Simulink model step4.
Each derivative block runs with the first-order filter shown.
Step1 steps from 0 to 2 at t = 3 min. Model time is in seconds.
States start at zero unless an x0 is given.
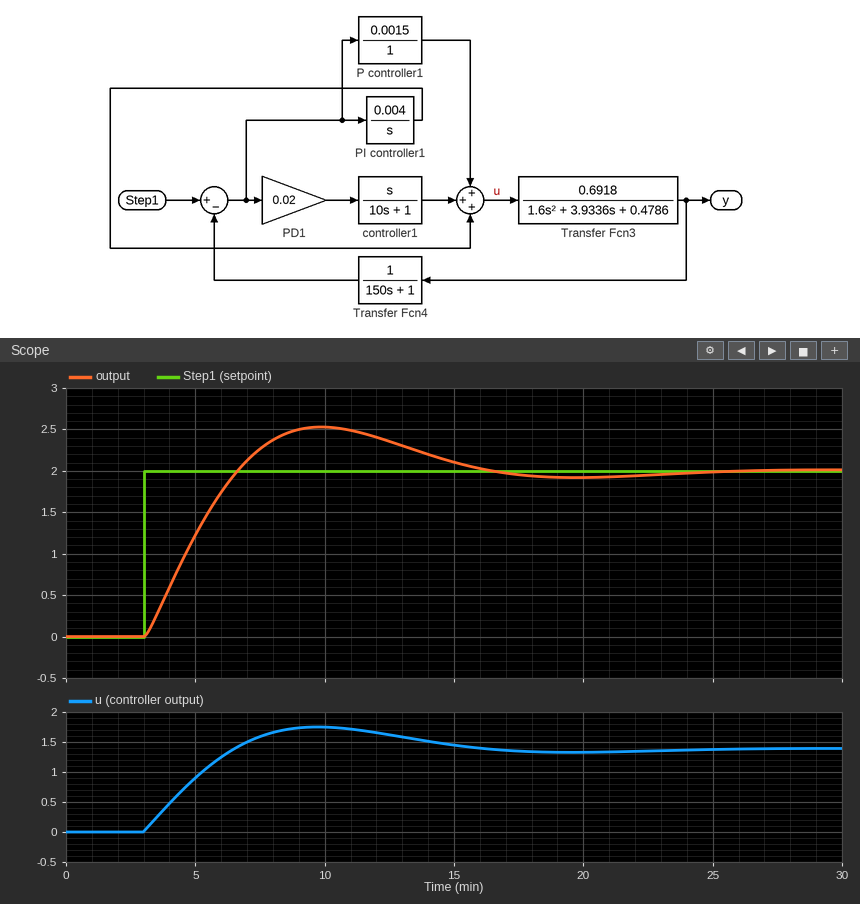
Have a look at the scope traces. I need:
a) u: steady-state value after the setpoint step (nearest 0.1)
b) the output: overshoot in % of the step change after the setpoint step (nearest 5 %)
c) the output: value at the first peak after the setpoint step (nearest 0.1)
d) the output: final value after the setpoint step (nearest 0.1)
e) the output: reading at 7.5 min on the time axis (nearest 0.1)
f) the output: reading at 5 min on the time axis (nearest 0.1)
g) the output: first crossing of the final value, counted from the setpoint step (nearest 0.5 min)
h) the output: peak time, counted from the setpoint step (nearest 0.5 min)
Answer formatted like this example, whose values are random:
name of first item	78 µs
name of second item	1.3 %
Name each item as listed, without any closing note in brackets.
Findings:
u: steady-state value after the setpoint step	1.4
the output: overshoot in % of the step change after the setpoint step	25 %
the output: value at the first peak after the setpoint step	2.5
the output: final value after the setpoint step	2.0
the output: reading at 7.5 min on the time axis	2.3
the output: reading at 5 min on the time axis	1.2
the output: first crossing of the final value, counted from the setpoint step	3.5 min
the output: peak time, counted from the setpoint step	7.0 min
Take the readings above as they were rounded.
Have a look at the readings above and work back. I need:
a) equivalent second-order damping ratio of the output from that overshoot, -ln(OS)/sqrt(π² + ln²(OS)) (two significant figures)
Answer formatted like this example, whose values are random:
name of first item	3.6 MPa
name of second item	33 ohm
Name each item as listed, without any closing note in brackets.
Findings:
equivalent second-order damping ratio of the output from that overshoot, -ln(OS)/sqrt(π² + ln²(OS))	0.40
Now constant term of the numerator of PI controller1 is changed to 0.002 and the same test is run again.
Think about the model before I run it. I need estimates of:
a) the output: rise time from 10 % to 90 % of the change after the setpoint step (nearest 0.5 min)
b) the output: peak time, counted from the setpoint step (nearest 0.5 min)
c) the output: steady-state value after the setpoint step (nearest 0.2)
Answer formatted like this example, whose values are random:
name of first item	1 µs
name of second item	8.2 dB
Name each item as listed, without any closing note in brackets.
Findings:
the output: rise time from 10 % to 90 % of the change after the setpoint step	6.5 min
the output: peak time, counted from the setpoint step	14.0 min
the output: steady-state value after the setpoint step	2.0
